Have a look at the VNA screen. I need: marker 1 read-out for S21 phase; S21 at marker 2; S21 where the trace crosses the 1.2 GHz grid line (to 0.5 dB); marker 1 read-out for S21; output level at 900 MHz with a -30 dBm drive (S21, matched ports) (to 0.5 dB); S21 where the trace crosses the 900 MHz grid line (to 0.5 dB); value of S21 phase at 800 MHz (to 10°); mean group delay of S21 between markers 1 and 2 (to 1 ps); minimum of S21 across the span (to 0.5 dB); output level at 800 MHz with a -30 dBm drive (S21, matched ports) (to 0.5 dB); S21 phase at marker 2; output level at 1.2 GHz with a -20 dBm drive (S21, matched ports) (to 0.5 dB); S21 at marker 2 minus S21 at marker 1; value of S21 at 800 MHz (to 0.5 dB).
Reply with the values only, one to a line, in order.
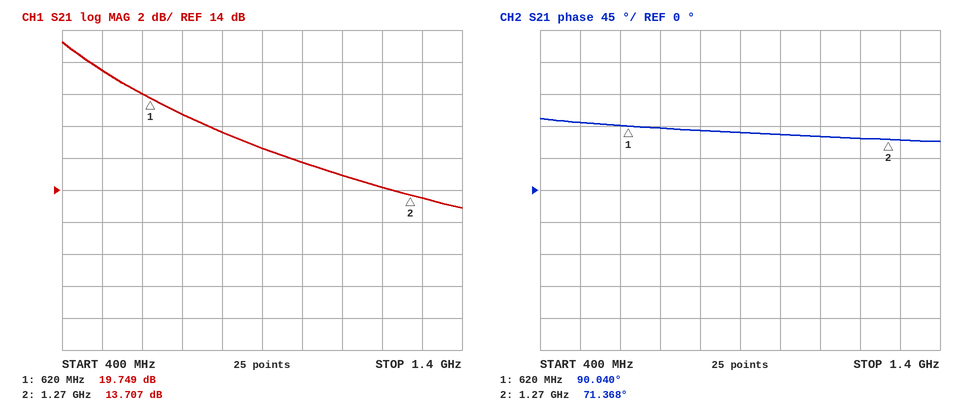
90.040°
13.707 dB
14.0 dB
19.749 dB
-13.5 dBm
16.5 dB
80°
80 ps
13.0 dB
-12.5 dBm
71.368°
-6.0 dBm
-6.042 dB
17.5 dB
